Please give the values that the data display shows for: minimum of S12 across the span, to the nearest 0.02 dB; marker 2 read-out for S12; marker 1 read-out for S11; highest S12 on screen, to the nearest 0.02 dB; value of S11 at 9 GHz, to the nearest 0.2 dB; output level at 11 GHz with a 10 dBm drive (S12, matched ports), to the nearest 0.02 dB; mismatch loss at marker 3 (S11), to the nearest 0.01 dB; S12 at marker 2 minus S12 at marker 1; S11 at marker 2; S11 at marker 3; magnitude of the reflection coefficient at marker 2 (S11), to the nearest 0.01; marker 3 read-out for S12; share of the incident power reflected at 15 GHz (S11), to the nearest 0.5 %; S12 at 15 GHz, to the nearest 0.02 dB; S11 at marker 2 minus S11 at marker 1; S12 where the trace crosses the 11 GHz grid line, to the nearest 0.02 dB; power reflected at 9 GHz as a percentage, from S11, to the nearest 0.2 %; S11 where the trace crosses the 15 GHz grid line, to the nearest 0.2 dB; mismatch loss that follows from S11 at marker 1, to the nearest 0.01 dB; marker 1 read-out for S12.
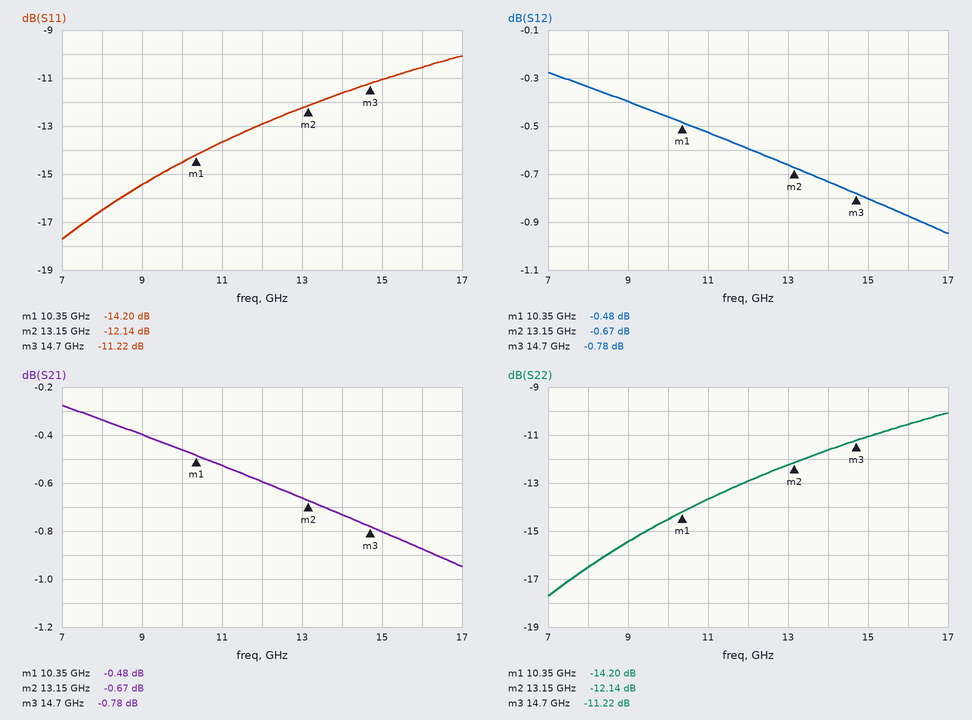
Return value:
-0.94 dB
-0.67 dB
-14.20 dB
-0.28 dB
-15.4 dB
9.48 dBm
0.34 dB
-0.19 dB
-12.14 dB
-11.22 dB
0.25
-0.78 dB
8.0 %
-0.80 dB
2.06 dB
-0.52 dB
2.8 %
-11.0 dB
0.17 dB
-0.48 dB
